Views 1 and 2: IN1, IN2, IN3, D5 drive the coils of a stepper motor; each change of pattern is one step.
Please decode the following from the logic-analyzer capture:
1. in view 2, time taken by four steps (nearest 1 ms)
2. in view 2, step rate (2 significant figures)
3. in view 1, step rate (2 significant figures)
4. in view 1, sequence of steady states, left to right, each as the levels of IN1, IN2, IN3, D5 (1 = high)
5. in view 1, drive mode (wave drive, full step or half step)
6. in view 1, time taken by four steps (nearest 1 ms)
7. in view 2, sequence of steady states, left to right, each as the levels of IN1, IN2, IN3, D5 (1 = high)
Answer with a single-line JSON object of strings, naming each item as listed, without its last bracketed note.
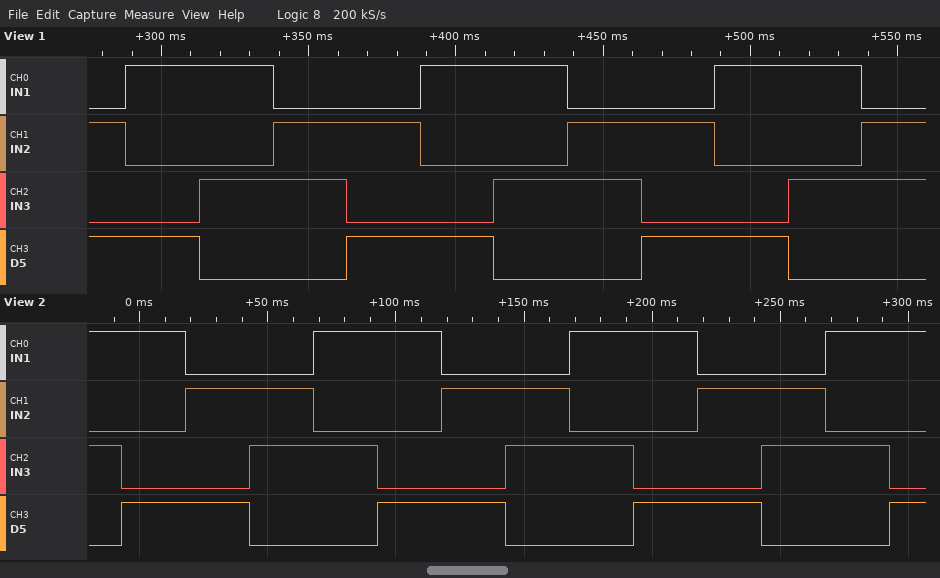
{"in view 2, time taken by four steps": "100 ms", "in view 2, step rate": "40 steps/s", "in view 1, step rate": "40 steps/s", "in view 1, sequence of steady states, left to right, each as the levels of IN1, IN2, IN3, D5": "0101 1001 1010 0110 0101 1001 1010 0110 0101 1001 1010 0110", "in view 1, drive mode": "full step", "in view 1, time taken by four steps": "100 ms", "in view 2, sequence of steady states, left to right, each as the levels of IN1, IN2, IN3, D5": "1010 1001 0101 0110 1010 1001 0101 0110 1010 1001 0101 0110 1010 1001"}
